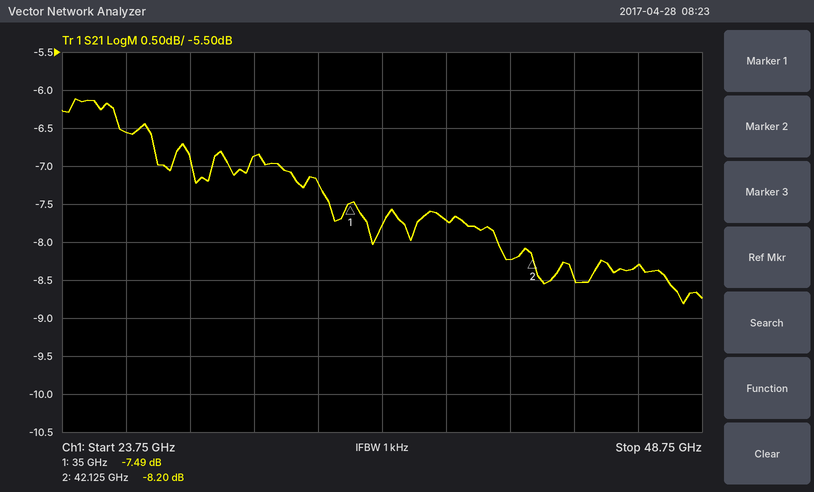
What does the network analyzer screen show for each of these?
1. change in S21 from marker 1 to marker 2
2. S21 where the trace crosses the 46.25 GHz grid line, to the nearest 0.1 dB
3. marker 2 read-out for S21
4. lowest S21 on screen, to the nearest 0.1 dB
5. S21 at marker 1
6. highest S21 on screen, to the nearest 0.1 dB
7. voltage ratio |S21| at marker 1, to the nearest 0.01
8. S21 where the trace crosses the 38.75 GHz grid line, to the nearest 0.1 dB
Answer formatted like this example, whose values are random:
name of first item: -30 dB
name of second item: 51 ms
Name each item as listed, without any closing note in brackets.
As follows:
change in S21 from marker 1 to marker 2: -0.71 dB
S21 where the trace crosses the 46.25 GHz grid line, to the nearest 0.1 dB: -8.3 dB
marker 2 read-out for S21: -8.20 dB
lowest S21 on screen, to the nearest 0.1 dB: -8.8 dB
S21 at marker 1: -7.49 dB
highest S21 on screen, to the nearest 0.1 dB: -6.1 dB
voltage ratio |S21| at marker 1, to the nearest 0.01: 0.42
S21 where the trace crosses the 38.75 GHz grid line, to the nearest 0.1 dB: -7.7 dB
